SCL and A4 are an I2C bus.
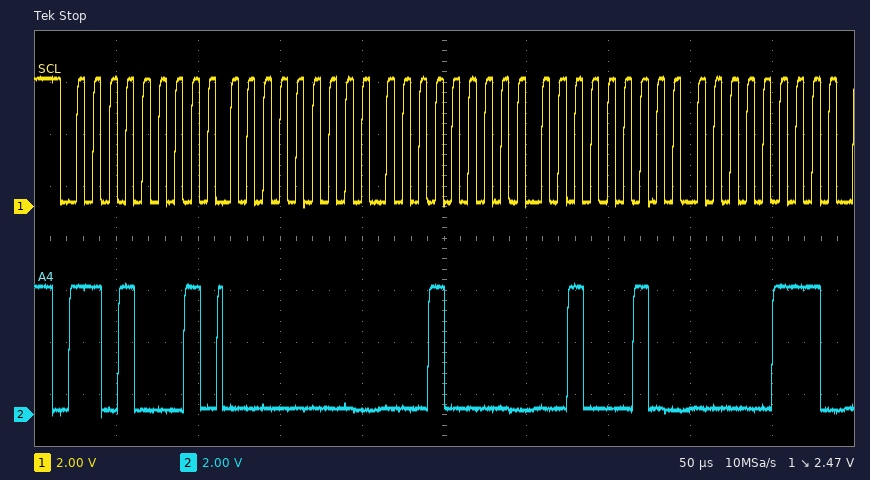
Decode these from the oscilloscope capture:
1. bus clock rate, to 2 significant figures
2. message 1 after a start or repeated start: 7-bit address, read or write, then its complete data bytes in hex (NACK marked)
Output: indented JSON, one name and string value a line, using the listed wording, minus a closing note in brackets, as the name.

{
  "bus clock rate, to 2 significant figures": "100 kHz",
  "message 1 after a start or repeated start: 7-bit address, read or write, then its complete data bytes in hex": "0x68 read: 00 10 22 07"
}
